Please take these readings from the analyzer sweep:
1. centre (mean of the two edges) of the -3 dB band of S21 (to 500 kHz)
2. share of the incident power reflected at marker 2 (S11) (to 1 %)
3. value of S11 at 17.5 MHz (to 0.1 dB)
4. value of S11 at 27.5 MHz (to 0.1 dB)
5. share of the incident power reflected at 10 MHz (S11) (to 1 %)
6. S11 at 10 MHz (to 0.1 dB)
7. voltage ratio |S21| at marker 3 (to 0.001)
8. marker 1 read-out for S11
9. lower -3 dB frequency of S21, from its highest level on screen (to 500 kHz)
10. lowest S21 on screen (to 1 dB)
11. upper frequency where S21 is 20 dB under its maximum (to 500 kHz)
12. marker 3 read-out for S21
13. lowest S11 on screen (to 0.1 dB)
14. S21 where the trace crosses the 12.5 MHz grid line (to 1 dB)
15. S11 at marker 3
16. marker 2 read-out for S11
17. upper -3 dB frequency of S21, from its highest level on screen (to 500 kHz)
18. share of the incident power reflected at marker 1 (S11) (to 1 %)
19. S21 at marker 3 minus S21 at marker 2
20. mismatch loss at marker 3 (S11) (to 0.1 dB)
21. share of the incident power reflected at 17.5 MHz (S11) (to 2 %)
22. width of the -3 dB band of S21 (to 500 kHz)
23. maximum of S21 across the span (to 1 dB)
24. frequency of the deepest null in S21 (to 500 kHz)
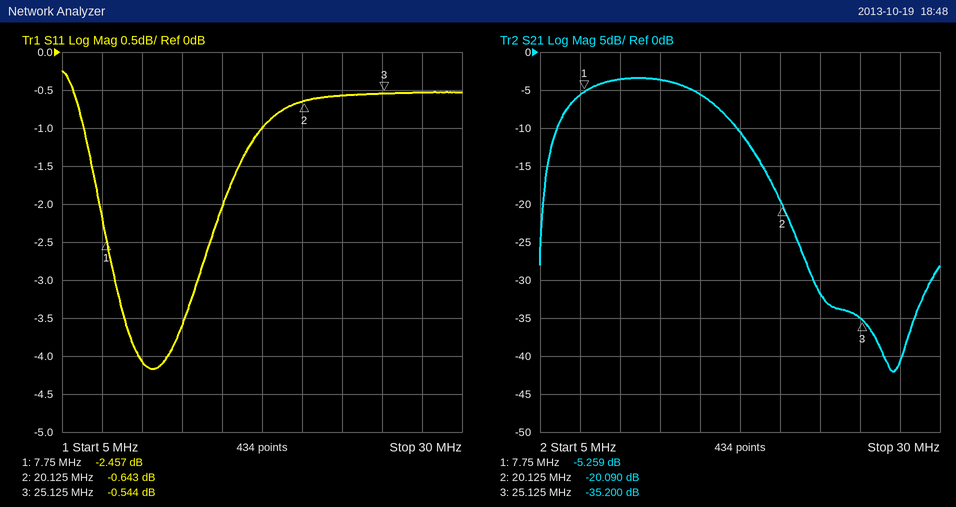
11.5 MHz
86 %
-1.0 dB
-0.5 dB
39 %
-4.1 dB
0.017
-2.457 dB
7.0 MHz
-42 dB
21.0 MHz
-35.200 dB
-4.2 dB
-4 dB
-0.544 dB
-0.643 dB
15.5 MHz
57 %
-15.110 dB
9.3 dB
80 %
8.5 MHz
-3 dB
27.0 MHz
